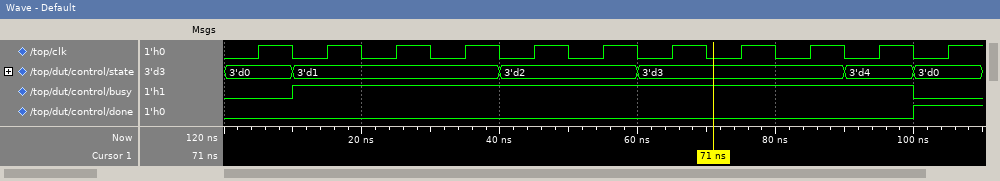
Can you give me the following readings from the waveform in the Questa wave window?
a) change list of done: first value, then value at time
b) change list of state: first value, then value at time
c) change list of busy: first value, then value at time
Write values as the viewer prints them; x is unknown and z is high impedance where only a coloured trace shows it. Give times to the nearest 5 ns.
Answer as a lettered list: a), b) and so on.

a) 0, 1 at 100 ns
b) 3'd0, 3'd1 at 10 ns, 3'd2 at 40 ns, 3'd3 at 60 ns, 3'd4 at 90 ns, 3'd0 at 100 ns
c) 0, 1 at 10 ns, 0 at 100 ns
